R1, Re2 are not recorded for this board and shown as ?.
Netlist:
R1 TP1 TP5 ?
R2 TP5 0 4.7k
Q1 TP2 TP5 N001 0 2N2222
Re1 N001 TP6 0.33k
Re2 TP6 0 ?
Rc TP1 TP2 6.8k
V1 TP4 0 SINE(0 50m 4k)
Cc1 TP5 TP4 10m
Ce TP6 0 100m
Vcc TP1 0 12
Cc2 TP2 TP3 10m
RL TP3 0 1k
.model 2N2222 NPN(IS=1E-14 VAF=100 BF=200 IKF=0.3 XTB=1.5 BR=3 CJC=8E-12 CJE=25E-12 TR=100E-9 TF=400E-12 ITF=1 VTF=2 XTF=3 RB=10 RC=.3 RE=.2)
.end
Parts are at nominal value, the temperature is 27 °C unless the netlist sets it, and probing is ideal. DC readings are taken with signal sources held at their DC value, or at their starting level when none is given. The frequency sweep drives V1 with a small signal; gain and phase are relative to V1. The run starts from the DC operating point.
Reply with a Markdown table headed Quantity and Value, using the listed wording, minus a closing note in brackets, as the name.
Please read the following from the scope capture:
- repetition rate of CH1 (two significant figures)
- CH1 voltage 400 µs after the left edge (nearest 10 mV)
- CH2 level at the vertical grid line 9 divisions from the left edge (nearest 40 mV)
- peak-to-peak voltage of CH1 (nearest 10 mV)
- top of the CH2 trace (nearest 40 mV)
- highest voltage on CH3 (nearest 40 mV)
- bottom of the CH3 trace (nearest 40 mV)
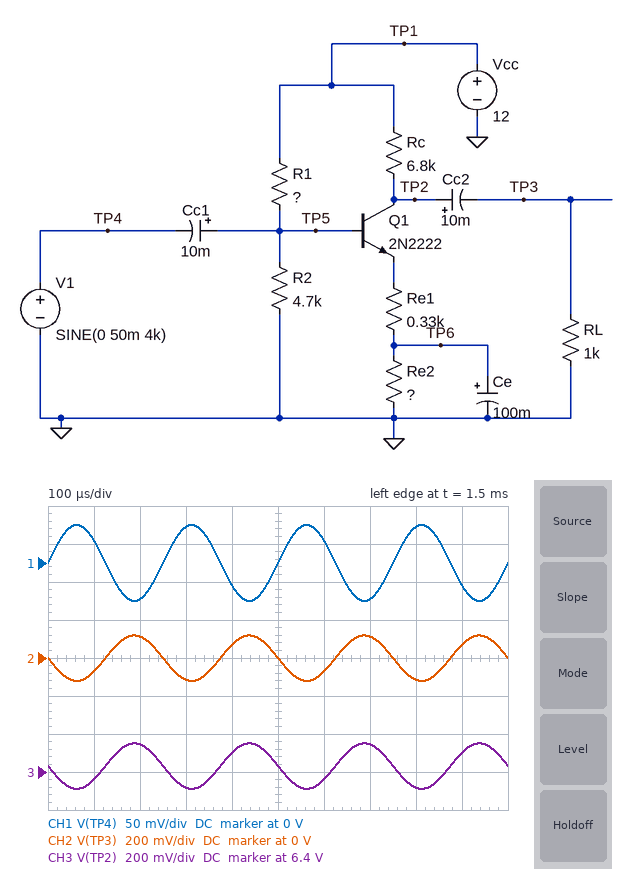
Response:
| Quantity | Value |
|---|---|
| repetition rate of CH1 | 4.0 kHz |
| CH1 voltage 400 µs after the left edge | -30 mV |
| CH2 level at the vertical grid line 9 divisions from the left edge | 80 mV |
| peak-to-peak voltage of CH1 | 100 mV |
| top of the CH2 trace | 120 mV |
| highest voltage on CH3 | 6.56 V |
| bottom of the CH3 trace | 6.32 V |
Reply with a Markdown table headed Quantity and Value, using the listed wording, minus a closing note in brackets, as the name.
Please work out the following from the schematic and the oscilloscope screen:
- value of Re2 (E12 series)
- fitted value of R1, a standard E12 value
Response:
| Quantity | Value |
|---|---|
| value of Re2 | 680 Ω |
| fitted value of R1, a standard E12 value | 33 kΩ |
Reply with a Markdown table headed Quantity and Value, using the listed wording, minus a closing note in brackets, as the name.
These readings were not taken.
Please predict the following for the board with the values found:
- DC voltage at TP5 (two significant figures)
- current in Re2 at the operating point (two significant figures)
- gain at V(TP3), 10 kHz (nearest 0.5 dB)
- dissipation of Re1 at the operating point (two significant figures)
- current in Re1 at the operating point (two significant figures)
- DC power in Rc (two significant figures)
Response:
| Quantity | Value |
|---|---|
| DC voltage at TP5 | 1.5 V |
| current in Re2 at the operating point | 820 µA |
| gain at V(TP3), 10 kHz | 7.5 dB |
| dissipation of Re1 at the operating point | 220 µW |
| current in Re1 at the operating point | 820 µA |
| DC power in Rc | 4.6 mW |
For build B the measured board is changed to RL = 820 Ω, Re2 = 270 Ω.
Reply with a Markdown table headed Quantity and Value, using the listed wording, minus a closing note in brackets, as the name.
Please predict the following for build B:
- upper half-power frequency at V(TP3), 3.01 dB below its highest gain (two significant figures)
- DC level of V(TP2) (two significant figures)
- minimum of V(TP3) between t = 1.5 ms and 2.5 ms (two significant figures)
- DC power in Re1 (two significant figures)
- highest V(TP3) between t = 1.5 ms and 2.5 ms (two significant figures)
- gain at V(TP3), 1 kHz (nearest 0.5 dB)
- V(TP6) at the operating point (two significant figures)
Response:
| Quantity | Value |
|---|---|
| upper half-power frequency at V(TP3), 3.01 dB below its highest gain | 67 MHz |
| DC level of V(TP2) | 2.9 V |
| minimum of V(TP3) between t = 1.5 ms and 2.5 ms | -100 mV |
| DC power in Re1 | 600 µW |
| highest V(TP3) between t = 1.5 ms and 2.5 ms | 100 mV |
| gain at V(TP3), 1 kHz | 6.5 dB |
| V(TP6) at the operating point | 360 mV |
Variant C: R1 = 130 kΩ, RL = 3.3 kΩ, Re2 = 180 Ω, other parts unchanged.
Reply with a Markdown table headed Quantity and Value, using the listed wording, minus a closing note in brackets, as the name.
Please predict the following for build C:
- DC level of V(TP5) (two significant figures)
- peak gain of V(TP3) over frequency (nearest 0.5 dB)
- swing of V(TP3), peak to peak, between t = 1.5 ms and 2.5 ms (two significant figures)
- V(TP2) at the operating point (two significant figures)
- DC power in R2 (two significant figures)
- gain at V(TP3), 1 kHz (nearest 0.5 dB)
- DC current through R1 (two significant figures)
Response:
| Quantity | Value |
|---|---|
| DC level of V(TP5) | 420 mV |
| peak gain of V(TP3) over frequency | -0.5 dB |
| swing of V(TP3), peak to peak, between t = 1.5 ms and 2.5 ms | 1.8 mV |
| V(TP2) at the operating point | 12 V |
| DC power in R2 | 37 µW |
| gain at V(TP3), 1 kHz | -40.0 dB |
| DC current through R1 | 89 µA |
